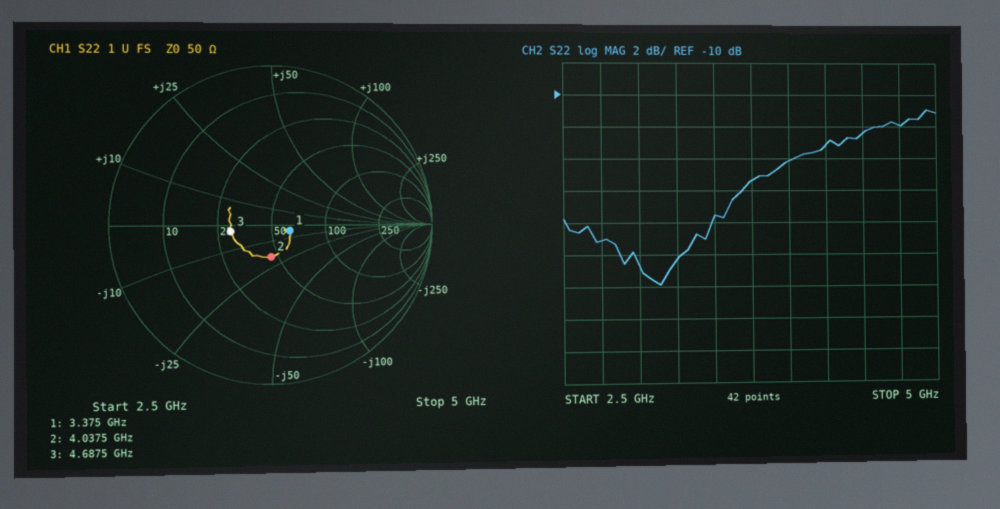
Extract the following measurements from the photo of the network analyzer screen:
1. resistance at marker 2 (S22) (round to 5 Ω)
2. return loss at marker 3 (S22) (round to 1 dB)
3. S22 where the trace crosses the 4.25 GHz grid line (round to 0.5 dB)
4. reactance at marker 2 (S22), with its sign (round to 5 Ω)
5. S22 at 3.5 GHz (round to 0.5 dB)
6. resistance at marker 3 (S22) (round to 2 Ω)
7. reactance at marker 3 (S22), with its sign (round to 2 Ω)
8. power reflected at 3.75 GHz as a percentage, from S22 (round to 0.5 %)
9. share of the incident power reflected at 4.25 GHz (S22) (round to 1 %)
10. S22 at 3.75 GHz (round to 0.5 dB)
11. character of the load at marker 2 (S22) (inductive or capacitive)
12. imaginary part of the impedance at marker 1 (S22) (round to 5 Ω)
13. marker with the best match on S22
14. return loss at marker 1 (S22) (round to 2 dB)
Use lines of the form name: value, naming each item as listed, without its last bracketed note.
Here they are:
resistance at marker 2 (S22): 45 Ω
return loss at marker 3 (S22): 12 dB
S22 where the trace crosses the 4.25 GHz grid line: -13.0 dB
reactance at marker 2 (S22), with its sign: -20 Ω
S22 at 3.5 GHz: -17.5 dB
resistance at marker 3 (S22): 30 Ω
reactance at marker 3 (S22), with its sign: -2 Ω
power reflected at 3.75 GHz as a percentage, from S22: 3.0 %
share of the incident power reflected at 4.25 GHz (S22): 5 %
S22 at 3.75 GHz: -15.5 dB
character of the load at marker 2 (S22): capacitive
imaginary part of the impedance at marker 1 (S22): -5 Ω
marker with the best match on S22: marker 1
return loss at marker 1 (S22): 18 dB
